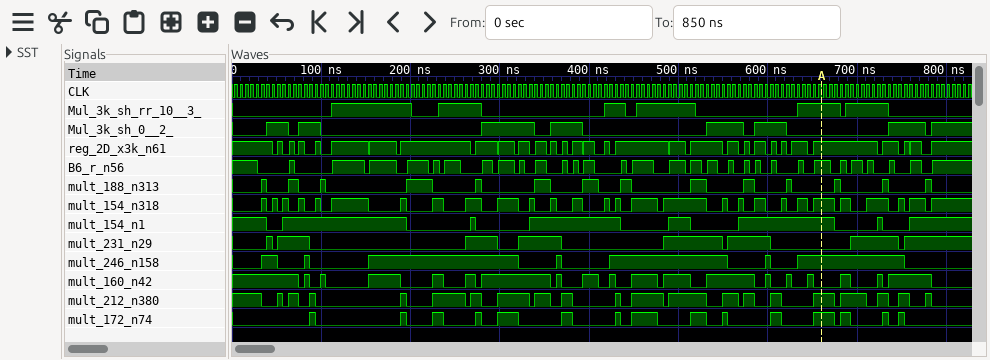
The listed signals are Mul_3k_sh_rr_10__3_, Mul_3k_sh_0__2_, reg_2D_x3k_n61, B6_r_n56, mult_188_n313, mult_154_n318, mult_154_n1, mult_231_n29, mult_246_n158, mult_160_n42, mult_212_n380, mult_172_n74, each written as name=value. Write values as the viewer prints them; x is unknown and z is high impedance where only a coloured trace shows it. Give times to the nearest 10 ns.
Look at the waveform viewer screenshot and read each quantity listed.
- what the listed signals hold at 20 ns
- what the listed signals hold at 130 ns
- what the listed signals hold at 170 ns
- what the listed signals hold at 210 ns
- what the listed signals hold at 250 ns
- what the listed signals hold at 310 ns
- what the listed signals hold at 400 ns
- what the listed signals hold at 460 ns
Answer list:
Mul_3k_sh_rr_10__3_=0, Mul_3k_sh_0__2_=0, reg_2D_x3k_n61=1, B6_r_n56=1, mult_188_n313=0, mult_154_n318=0, mult_154_n1=1, mult_231_n29=0, mult_246_n158=0, mult_160_n42=1, mult_212_n380=1, mult_172_n74=0
Mul_3k_sh_rr_10__3_=1, Mul_3k_sh_0__2_=0, reg_2D_x3k_n61=1, B6_r_n56=1, mult_188_n313=0, mult_154_n318=1, mult_154_n1=1, mult_231_n29=0, mult_246_n158=0, mult_160_n42=0, mult_212_n380=0, mult_172_n74=0
Mul_3k_sh_rr_10__3_=1, Mul_3k_sh_0__2_=0, reg_2D_x3k_n61=1, B6_r_n56=1, mult_188_n313=0, mult_154_n318=0, mult_154_n1=1, mult_231_n29=0, mult_246_n158=1, mult_160_n42=1, mult_212_n380=0, mult_172_n74=0
Mul_3k_sh_rr_10__3_=0, Mul_3k_sh_0__2_=0, reg_2D_x3k_n61=1, B6_r_n56=1, mult_188_n313=1, mult_154_n318=0, mult_154_n1=0, mult_231_n29=0, mult_246_n158=1, mult_160_n42=0, mult_212_n380=0, mult_172_n74=0
Mul_3k_sh_rr_10__3_=1, Mul_3k_sh_0__2_=0, reg_2D_x3k_n61=1, B6_r_n56=1, mult_188_n313=0, mult_154_n318=0, mult_154_n1=0, mult_231_n29=0, mult_246_n158=1, mult_160_n42=0, mult_212_n380=1, mult_172_n74=0
Mul_3k_sh_rr_10__3_=0, Mul_3k_sh_0__2_=1, reg_2D_x3k_n61=1, B6_r_n56=1, mult_188_n313=0, mult_154_n318=1, mult_154_n1=0, mult_231_n29=0, mult_246_n158=1, mult_160_n42=1, mult_212_n380=1, mult_172_n74=1
Mul_3k_sh_rr_10__3_=0, Mul_3k_sh_0__2_=0, reg_2D_x3k_n61=1, B6_r_n56=1, mult_188_n313=1, mult_154_n318=0, mult_154_n1=1, mult_231_n29=0, mult_246_n158=0, mult_160_n42=1, mult_212_n380=0, mult_172_n74=0
Mul_3k_sh_rr_10__3_=1, Mul_3k_sh_0__2_=0, reg_2D_x3k_n61=1, B6_r_n56=1, mult_188_n313=0, mult_154_n318=1, mult_154_n1=0, mult_231_n29=0, mult_246_n158=1, mult_160_n42=1, mult_212_n380=1, mult_172_n74=1
